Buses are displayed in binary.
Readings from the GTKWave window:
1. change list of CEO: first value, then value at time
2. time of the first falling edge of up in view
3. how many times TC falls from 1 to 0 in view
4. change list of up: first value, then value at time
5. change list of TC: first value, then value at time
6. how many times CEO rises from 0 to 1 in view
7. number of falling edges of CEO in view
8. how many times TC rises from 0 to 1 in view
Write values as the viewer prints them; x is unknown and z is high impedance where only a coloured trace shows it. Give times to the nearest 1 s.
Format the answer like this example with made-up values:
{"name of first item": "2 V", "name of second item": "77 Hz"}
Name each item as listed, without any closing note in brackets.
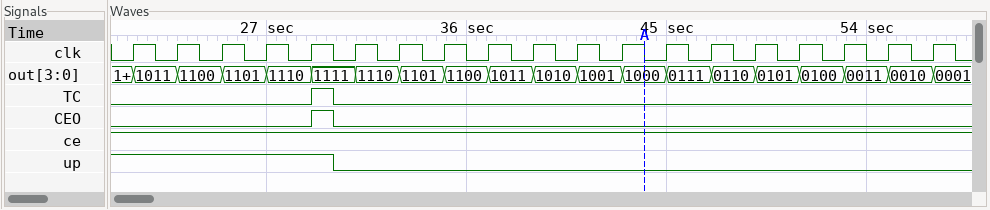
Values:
{"change list of CEO: first value, then value at time": "0, 1 at 29 s, 0 at 30 s", "time of the first falling edge of up in view": "30 s", "how many times TC falls from 1 to 0 in view": "1", "change list of up: first value, then value at time": "1, 0 at 30 s", "change list of TC: first value, then value at time": "0, 1 at 29 s, 0 at 30 s", "how many times CEO rises from 0 to 1 in view": "1", "number of falling edges of CEO in view": "1", "how many times TC rises from 0 to 1 in view": "1"}
